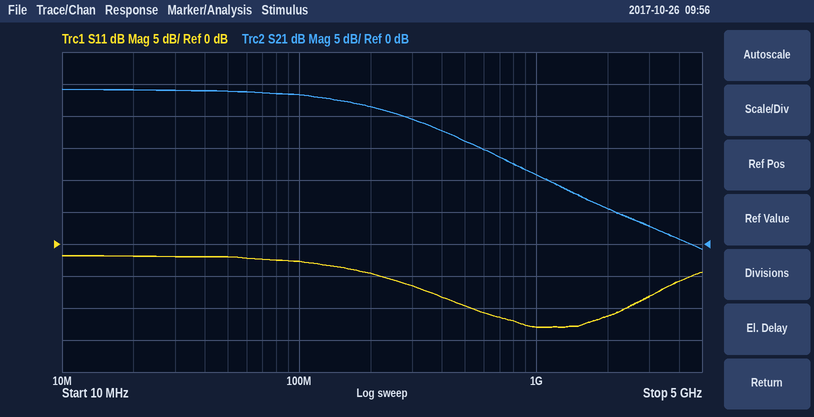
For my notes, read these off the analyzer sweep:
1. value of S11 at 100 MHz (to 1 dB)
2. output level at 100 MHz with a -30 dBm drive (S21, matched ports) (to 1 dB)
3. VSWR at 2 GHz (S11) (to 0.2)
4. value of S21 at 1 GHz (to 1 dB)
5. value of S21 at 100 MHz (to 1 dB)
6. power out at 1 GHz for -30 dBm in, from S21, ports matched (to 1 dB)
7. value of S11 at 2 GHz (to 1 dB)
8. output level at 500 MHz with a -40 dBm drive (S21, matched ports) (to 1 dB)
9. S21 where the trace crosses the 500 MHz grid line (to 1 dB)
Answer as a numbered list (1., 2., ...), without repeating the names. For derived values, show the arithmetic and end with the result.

1. -3 dB
2. -30 dBm + (23 dB) = -7 dBm
3. |Γ| = 10^(-11/20) = 0.2818; VSWR = (1 + 0.2818)/(1 − 0.2818) ≈ 1.8
4. 11 dB
5. 23 dB
6. -30 dBm + (11 dB) = -19 dBm
7. -11 dB
8. -40 dBm + (16 dB) = -24 dBm
9. 16 dB
